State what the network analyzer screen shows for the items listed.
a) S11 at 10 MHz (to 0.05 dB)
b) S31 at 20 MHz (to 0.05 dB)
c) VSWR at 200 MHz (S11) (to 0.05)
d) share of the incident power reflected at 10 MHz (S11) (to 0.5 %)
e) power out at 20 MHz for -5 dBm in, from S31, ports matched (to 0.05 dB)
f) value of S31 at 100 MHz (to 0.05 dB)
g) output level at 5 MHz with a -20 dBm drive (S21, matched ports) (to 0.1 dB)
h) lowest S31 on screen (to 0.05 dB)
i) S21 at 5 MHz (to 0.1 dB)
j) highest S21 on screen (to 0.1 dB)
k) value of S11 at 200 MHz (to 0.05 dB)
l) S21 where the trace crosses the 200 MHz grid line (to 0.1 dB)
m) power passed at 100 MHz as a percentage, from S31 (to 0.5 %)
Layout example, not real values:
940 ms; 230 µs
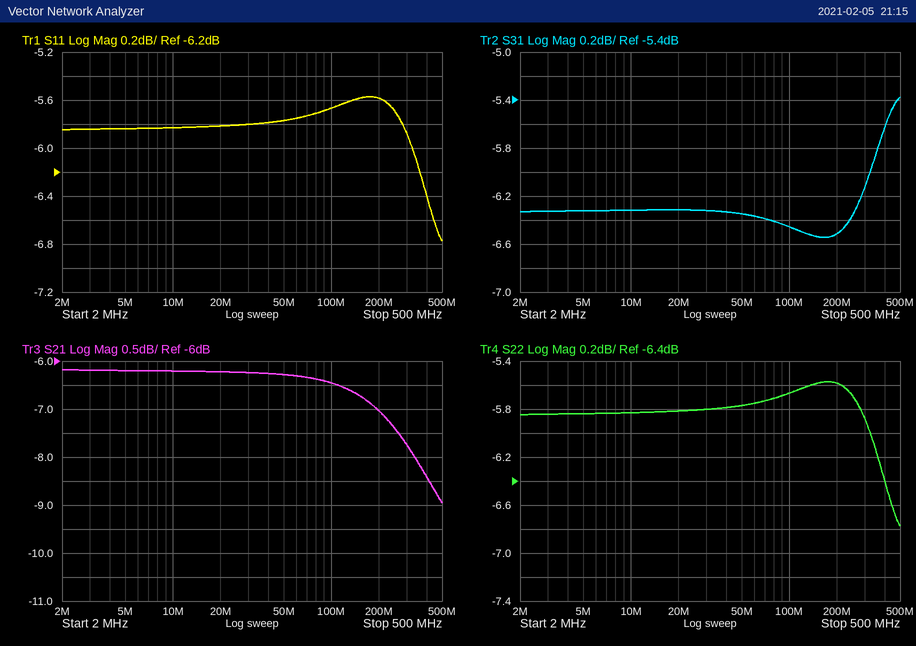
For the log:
-5.85 dB; -6.30 dB; 3.20; 26.0 %; -11.30 dBm; -6.45 dB; -26.2 dBm; -6.55 dB; -6.2 dB; -6.2 dB; -5.60 dB; -7.0 dB; 22.5 %
